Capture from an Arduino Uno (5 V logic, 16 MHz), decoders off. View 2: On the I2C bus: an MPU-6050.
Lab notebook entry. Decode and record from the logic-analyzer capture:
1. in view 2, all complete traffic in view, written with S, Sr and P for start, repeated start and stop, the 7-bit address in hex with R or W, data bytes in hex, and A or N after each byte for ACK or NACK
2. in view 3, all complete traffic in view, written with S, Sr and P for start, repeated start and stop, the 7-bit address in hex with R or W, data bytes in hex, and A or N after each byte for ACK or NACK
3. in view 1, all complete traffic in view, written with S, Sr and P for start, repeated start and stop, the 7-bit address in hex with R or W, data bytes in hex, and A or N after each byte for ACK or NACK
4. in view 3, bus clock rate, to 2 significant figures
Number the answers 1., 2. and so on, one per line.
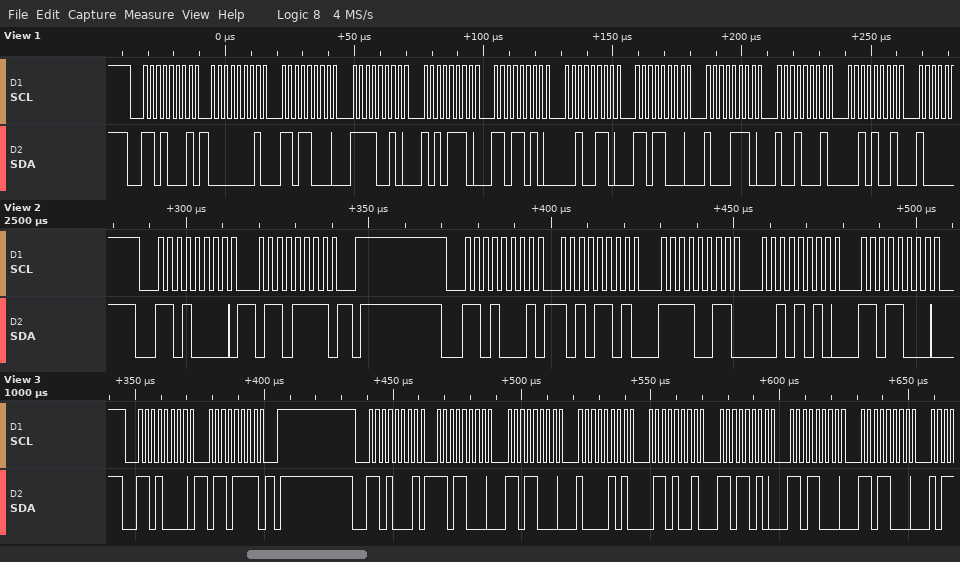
1. S 68W A 6F A P S 68R A AD A F3 A 2A A D8 A
2. S 68W A 6F A P S 68R A D8 A D8 A 85 A 69 A DA A D8 A D8 A
3. S 68R A 01 A D8 A F2 A AE A DA A 26 A D8 A 8E A 91 A 29 A
4. 400 kHz
